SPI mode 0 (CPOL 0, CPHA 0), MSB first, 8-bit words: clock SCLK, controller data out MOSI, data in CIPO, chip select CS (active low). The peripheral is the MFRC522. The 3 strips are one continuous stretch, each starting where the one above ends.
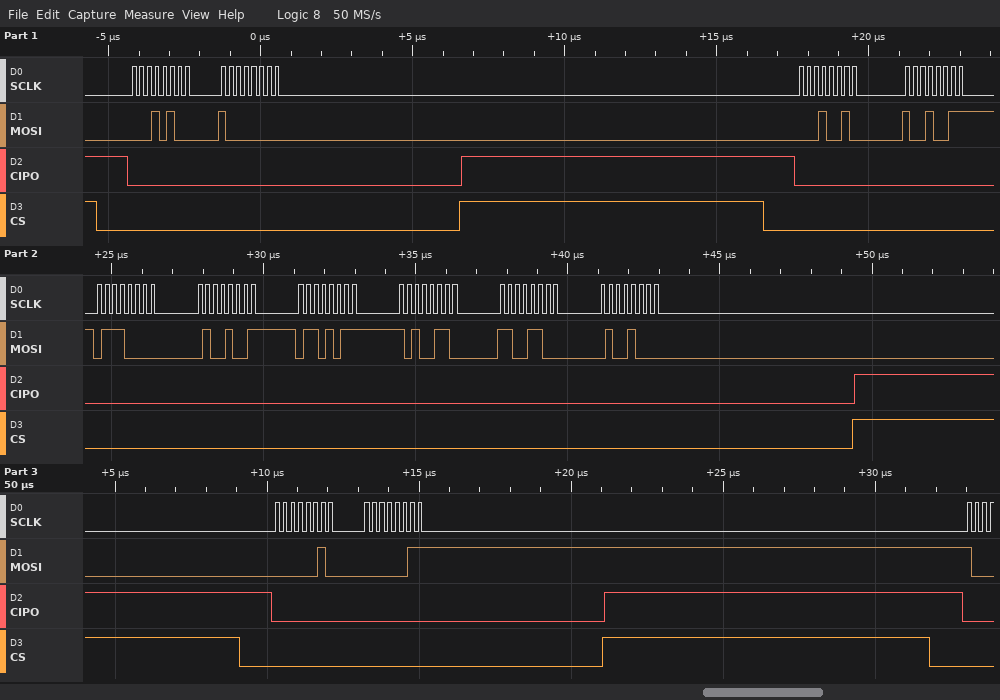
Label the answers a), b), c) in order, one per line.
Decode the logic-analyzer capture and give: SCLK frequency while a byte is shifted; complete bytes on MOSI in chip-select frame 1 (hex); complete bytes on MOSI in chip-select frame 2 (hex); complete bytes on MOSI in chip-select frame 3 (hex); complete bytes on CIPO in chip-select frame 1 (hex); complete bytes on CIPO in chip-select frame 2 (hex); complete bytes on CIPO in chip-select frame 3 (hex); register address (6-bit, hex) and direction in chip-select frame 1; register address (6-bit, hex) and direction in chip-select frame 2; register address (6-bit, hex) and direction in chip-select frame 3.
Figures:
a) 4 MHz
b) 14 80
c) 12 93 70 49 6B A6 CC 48
d) 02 03
e) 00 00
f) 00 00 00 00 00 00 00 00
g) 00 00
h) 0x0A write
i) 0x09 write
j) 0x01 write
